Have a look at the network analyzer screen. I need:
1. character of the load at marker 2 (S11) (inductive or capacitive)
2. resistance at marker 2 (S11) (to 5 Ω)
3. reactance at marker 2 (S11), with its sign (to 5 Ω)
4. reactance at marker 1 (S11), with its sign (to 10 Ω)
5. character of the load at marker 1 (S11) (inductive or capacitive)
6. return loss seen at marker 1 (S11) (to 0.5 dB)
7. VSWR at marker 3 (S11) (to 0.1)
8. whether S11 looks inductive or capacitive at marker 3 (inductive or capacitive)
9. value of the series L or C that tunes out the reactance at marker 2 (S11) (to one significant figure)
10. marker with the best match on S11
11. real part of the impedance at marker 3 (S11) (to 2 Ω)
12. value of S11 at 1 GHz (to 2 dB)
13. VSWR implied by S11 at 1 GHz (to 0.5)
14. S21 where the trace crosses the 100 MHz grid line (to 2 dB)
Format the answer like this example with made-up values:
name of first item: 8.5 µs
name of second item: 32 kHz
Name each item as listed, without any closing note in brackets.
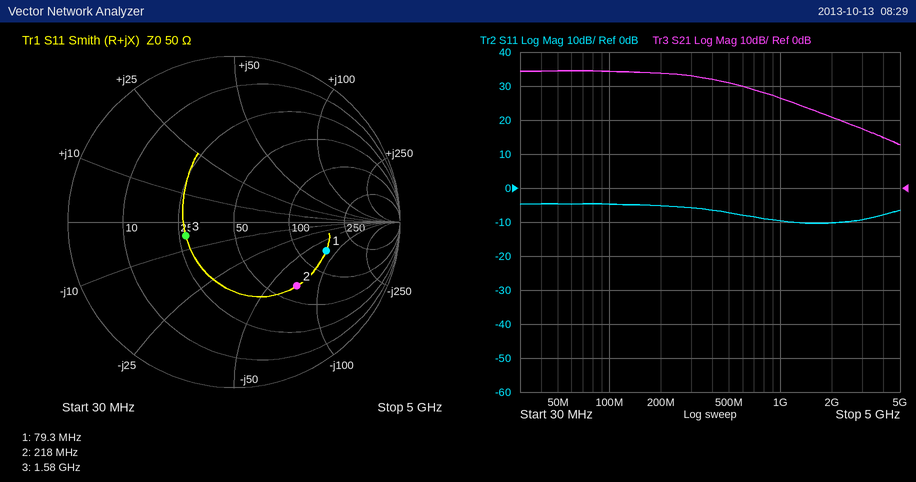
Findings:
character of the load at marker 2 (S11): capacitive
resistance at marker 2 (S11): 65 Ω
reactance at marker 2 (S11), with its sign: -70 Ω
reactance at marker 1 (S11), with its sign: -80 Ω
character of the load at marker 1 (S11): capacitive
return loss seen at marker 1 (S11): 4.5 dB
VSWR at marker 3 (S11): 1.9
whether S11 looks inductive or capacitive at marker 3: capacitive
value of the series L or C that tunes out the reactance at marker 2 (S11): 50 nH
marker with the best match on S11: marker 3
real part of the impedance at marker 3 (S11): 28 Ω
value of S11 at 1 GHz: -10 dB
VSWR implied by S11 at 1 GHz: 2.0
S21 where the trace crosses the 100 MHz grid line: 34 dB
